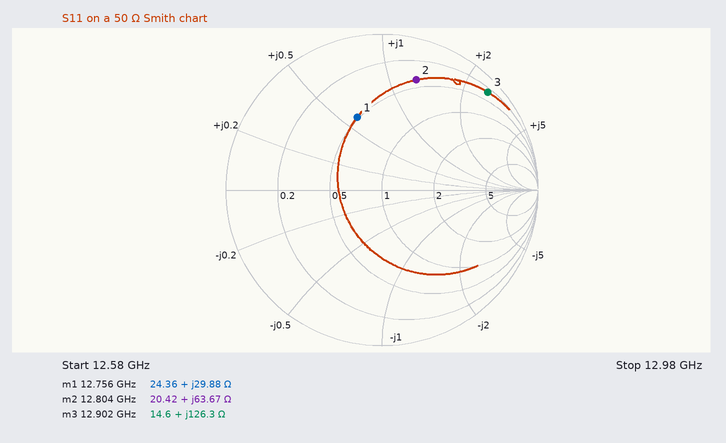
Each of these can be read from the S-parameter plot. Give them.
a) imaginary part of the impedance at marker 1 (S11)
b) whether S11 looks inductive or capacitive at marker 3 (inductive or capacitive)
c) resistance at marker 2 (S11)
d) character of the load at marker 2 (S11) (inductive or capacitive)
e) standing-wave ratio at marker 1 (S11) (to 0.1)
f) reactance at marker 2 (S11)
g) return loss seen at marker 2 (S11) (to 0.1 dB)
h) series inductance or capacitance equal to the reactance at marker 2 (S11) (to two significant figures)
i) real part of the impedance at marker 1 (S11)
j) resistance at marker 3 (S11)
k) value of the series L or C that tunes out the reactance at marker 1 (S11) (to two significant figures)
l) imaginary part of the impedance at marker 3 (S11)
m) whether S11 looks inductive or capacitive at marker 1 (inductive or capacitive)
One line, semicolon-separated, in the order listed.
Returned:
+29.88 Ω; inductive; 20.42 Ω; inductive; 2.9; +63.67 Ω; 2.6 dB; 790 pH; 24.36 Ω; 14.6 Ω; 420 fF; +126.3 Ω; inductive
